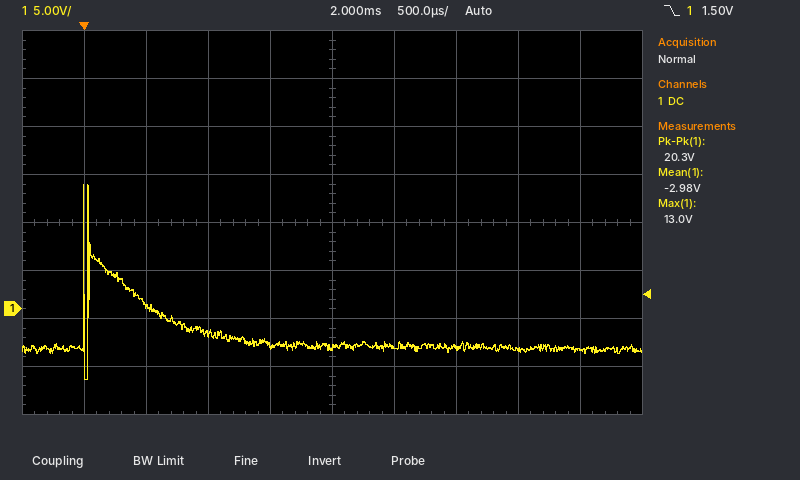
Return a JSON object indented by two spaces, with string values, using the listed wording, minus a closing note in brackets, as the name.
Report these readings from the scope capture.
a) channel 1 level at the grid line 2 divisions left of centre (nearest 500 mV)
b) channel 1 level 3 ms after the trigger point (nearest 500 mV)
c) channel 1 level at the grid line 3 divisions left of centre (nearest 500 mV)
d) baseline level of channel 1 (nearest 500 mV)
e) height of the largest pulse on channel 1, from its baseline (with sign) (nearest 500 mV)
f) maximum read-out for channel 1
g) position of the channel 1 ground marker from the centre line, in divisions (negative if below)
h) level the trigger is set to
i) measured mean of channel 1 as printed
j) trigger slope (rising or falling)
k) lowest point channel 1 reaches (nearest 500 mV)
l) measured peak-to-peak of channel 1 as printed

{
  "channel 1 level at the grid line 2 divisions left of centre": "-2.5 V",
  "channel 1 level 3 ms after the trigger point": "-4.0 V",
  "channel 1 level at the grid line 3 divisions left of centre": "500 mV",
  "baseline level of channel 1": "-4.0 V",
  "height of the largest pulse on channel 1, from its baseline (with sign)": "+17.0 V",
  "maximum read-out for channel 1": "13.0 V",
  "position of the channel 1 ground marker from the centre line, in divisions": "-1.8 div",
  "level the trigger is set to": "1.50 V",
  "measured mean of channel 1 as printed": "-2.98 V",
  "trigger slope": "falling",
  "lowest point channel 1 reaches": "-7.5 V",
  "measured peak-to-peak of channel 1 as printed": "20.3 V"
}
